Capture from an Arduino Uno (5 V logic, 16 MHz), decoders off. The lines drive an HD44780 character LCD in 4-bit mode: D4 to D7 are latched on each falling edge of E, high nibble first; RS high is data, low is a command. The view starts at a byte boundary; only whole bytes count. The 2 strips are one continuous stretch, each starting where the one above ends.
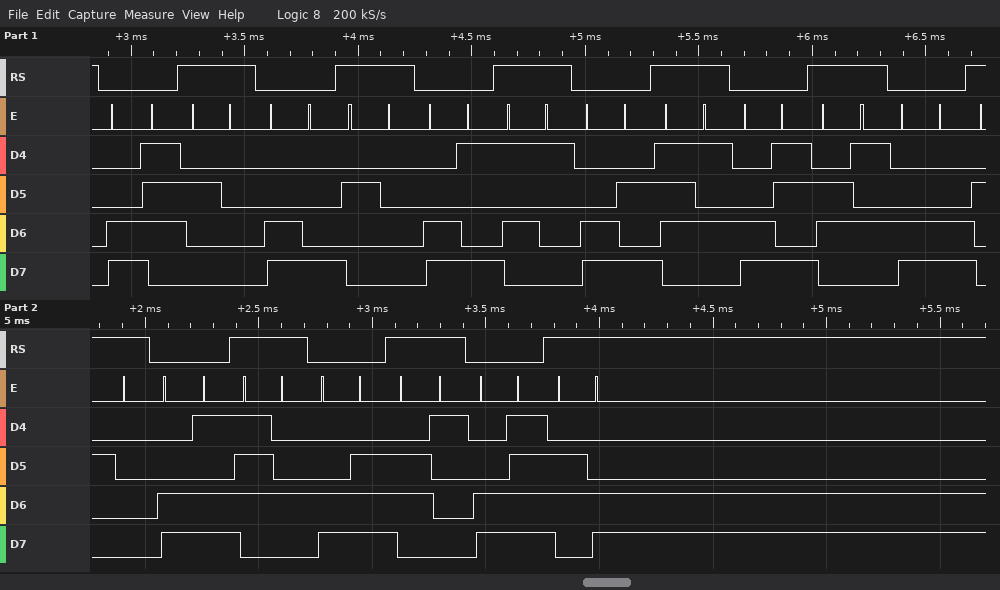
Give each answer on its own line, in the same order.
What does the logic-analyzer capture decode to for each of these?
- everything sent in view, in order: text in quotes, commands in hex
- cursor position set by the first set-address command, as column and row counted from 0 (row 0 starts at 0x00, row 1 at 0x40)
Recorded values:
0xC7 " " 0xC8 " " 0xC9 "Q" 0xCA "u" 0xCB "e" 0xCC " " 0xCD "t" 0xCE "a" 0xCF "l"
column 7, row 1
